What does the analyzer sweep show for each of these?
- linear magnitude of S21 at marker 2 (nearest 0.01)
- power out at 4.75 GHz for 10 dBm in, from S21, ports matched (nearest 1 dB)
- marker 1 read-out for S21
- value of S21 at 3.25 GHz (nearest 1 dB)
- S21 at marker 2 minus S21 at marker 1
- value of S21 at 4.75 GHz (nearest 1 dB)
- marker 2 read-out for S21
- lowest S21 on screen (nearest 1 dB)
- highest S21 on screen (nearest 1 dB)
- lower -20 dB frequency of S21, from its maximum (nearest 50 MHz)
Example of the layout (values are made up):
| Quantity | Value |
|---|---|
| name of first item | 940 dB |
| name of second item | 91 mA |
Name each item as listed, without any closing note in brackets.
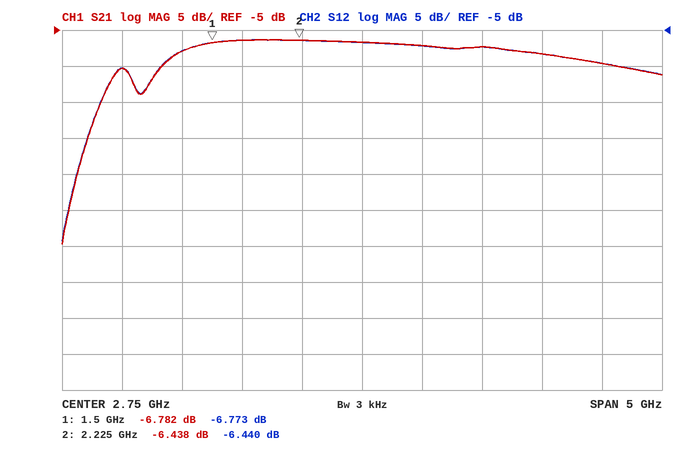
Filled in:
| Quantity | Value |
|---|---|
| linear magnitude of S21 at marker 2 | 0.48 |
| power out at 4.75 GHz for 10 dBm in, from S21, ports matched | 0 dBm |
| marker 1 read-out for S21 | -6.782 dB |
| value of S21 at 3.25 GHz | -7 dB |
| S21 at marker 2 minus S21 at marker 1 | 0.344 dB |
| value of S21 at 4.75 GHz | -10 dB |
| marker 2 read-out for S21 | -6.438 dB |
| lowest S21 on screen | -35 dB |
| highest S21 on screen | -6 dB |
| lower -20 dB frequency of S21, from its maximum | 350 MHz |
